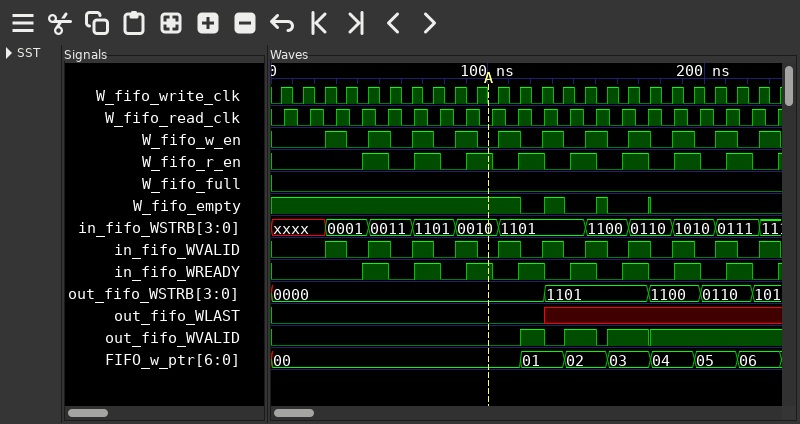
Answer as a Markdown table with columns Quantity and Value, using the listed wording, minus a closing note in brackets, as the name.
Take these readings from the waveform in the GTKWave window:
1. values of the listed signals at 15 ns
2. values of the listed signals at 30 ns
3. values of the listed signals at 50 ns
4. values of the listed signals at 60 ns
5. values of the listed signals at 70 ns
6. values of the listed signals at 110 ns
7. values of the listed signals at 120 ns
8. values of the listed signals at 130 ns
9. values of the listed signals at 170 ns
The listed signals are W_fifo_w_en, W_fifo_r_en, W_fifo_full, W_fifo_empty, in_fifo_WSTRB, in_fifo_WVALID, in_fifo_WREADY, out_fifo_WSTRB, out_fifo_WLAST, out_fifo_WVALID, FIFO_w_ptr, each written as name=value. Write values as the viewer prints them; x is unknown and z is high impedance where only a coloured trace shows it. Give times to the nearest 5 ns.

| Quantity | Value |
|---|---|
| values of the listed signals at 15 ns | W_fifo_w_en=0, W_fifo_r_en=0, W_fifo_full=0, W_fifo_empty=1, in_fifo_WSTRB=xxxx, in_fifo_WVALID=0, in_fifo_WREADY=0, out_fifo_WSTRB=0000, out_fifo_WLAST=0, out_fifo_WVALID=0, FIFO_w_ptr=00 |
| values of the listed signals at 30 ns | W_fifo_w_en=1, W_fifo_r_en=0, W_fifo_full=0, W_fifo_empty=1, in_fifo_WSTRB=0001, in_fifo_WVALID=1, in_fifo_WREADY=0, out_fifo_WSTRB=0000, out_fifo_WLAST=0, out_fifo_WVALID=0, FIFO_w_ptr=00 |
| values of the listed signals at 50 ns | W_fifo_w_en=1, W_fifo_r_en=1, W_fifo_full=0, W_fifo_empty=1, in_fifo_WSTRB=0011, in_fifo_WVALID=1, in_fifo_WREADY=1, out_fifo_WSTRB=0000, out_fifo_WLAST=0, out_fifo_WVALID=0, FIFO_w_ptr=00 |
| values of the listed signals at 60 ns | W_fifo_w_en=0, W_fifo_r_en=0, W_fifo_full=0, W_fifo_empty=1, in_fifo_WSTRB=0011, in_fifo_WVALID=0, in_fifo_WREADY=0, out_fifo_WSTRB=0000, out_fifo_WLAST=0, out_fifo_WVALID=0, FIFO_w_ptr=00 |
| values of the listed signals at 70 ns | W_fifo_w_en=1, W_fifo_r_en=1, W_fifo_full=0, W_fifo_empty=1, in_fifo_WSTRB=1101, in_fifo_WVALID=1, in_fifo_WREADY=1, out_fifo_WSTRB=0000, out_fifo_WLAST=0, out_fifo_WVALID=0, FIFO_w_ptr=00 |
| values of the listed signals at 110 ns | W_fifo_w_en=1, W_fifo_r_en=0, W_fifo_full=0, W_fifo_empty=1, in_fifo_WSTRB=1101, in_fifo_WVALID=1, in_fifo_WREADY=0, out_fifo_WSTRB=0000, out_fifo_WLAST=0, out_fifo_WVALID=0, FIFO_w_ptr=00 |
| values of the listed signals at 120 ns | W_fifo_w_en=0, W_fifo_r_en=1, W_fifo_full=0, W_fifo_empty=0, in_fifo_WSTRB=1101, in_fifo_WVALID=0, in_fifo_WREADY=1, out_fifo_WSTRB=0000, out_fifo_WLAST=0, out_fifo_WVALID=1, FIFO_w_ptr=01 |
| values of the listed signals at 130 ns | W_fifo_w_en=1, W_fifo_r_en=0, W_fifo_full=0, W_fifo_empty=1, in_fifo_WSTRB=1101, in_fifo_WVALID=1, in_fifo_WREADY=0, out_fifo_WSTRB=1101, out_fifo_WLAST=x, out_fifo_WVALID=0, FIFO_w_ptr=01 |
| values of the listed signals at 170 ns | W_fifo_w_en=1, W_fifo_r_en=1, W_fifo_full=0, W_fifo_empty=0, in_fifo_WSTRB=0110, in_fifo_WVALID=1, in_fifo_WREADY=1, out_fifo_WSTRB=1101, out_fifo_WLAST=x, out_fifo_WVALID=1, FIFO_w_ptr=03 |
